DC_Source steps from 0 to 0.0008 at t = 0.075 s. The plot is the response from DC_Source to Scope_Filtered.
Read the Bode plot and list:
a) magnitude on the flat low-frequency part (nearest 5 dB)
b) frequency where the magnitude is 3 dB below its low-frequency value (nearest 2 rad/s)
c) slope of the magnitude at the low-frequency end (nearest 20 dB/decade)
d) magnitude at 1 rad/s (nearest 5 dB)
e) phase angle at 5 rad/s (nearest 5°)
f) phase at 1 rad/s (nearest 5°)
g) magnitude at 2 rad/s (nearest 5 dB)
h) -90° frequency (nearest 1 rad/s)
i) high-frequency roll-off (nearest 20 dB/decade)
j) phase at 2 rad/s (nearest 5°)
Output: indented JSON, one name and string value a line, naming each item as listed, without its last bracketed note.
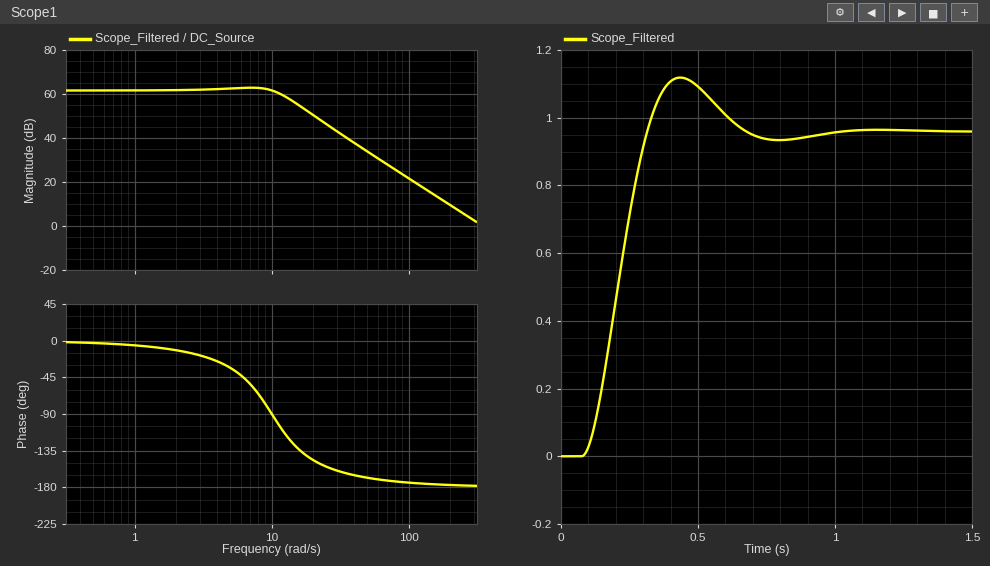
{
  "magnitude on the flat low-frequency part": "60 dB",
  "frequency where the magnitude is 3 dB below its low-frequency value": "12 rad/s",
  "slope of the magnitude at the low-frequency end": "0 dB/decade",
  "magnitude at 1 rad/s": "60 dB",
  "phase angle at 5 rad/s": "-35°",
  "phase at 1 rad/s": "-5°",
  "magnitude at 2 rad/s": "60 dB",
  "-90° frequency": "10 rad/s",
  "high-frequency roll-off": "-40 dB/decade",
  "phase at 2 rad/s": "-10°"
}
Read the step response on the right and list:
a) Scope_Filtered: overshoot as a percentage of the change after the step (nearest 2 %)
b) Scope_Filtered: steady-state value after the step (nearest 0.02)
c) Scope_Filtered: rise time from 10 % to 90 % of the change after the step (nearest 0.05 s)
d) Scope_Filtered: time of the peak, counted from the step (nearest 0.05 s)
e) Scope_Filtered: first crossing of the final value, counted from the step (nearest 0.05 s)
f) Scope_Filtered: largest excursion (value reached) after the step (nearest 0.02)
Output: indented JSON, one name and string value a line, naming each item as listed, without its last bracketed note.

{
  "Scope_Filtered: overshoot as a percentage of the change after the step": "16 %",
  "Scope_Filtered: steady-state value after the step": "0.96",
  "Scope_Filtered: rise time from 10 % to 90 % of the change after the step": "0.15 s",
  "Scope_Filtered: time of the peak, counted from the step": "0.35 s",
  "Scope_Filtered: first crossing of the final value, counted from the step": "0.25 s",
  "Scope_Filtered: largest excursion (value reached) after the step": "1.12"
}
